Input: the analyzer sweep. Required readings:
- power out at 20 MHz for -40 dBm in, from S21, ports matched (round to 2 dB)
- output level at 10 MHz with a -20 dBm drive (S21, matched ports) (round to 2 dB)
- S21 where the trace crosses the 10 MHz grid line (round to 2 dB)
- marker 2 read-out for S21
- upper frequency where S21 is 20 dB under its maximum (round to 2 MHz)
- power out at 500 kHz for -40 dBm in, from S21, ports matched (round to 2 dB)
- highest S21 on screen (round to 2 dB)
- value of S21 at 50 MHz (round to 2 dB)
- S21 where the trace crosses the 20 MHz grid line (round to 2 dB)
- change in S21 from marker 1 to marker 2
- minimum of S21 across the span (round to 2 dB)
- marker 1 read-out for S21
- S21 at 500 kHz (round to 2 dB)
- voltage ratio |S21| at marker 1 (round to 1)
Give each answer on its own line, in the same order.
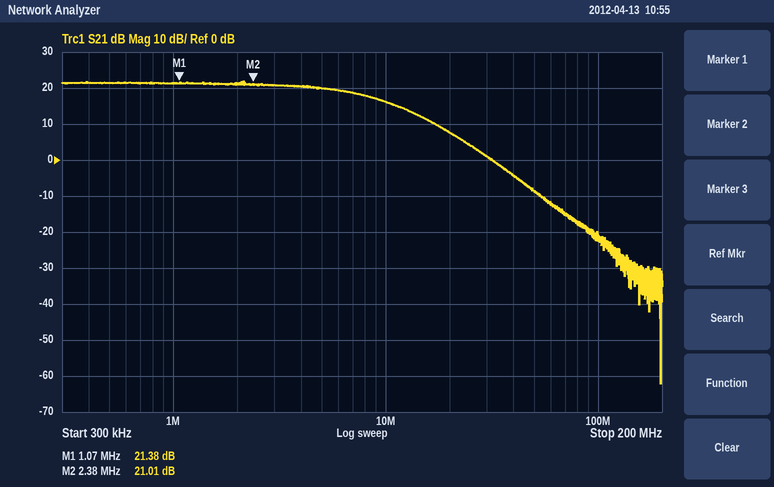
-32 dBm
-4 dBm
16 dB
21.01 dB
28 MHz
-18 dBm
22 dB
-8 dB
8 dB
-0.37 dB
-62 dB
21.38 dB
22 dB
12
